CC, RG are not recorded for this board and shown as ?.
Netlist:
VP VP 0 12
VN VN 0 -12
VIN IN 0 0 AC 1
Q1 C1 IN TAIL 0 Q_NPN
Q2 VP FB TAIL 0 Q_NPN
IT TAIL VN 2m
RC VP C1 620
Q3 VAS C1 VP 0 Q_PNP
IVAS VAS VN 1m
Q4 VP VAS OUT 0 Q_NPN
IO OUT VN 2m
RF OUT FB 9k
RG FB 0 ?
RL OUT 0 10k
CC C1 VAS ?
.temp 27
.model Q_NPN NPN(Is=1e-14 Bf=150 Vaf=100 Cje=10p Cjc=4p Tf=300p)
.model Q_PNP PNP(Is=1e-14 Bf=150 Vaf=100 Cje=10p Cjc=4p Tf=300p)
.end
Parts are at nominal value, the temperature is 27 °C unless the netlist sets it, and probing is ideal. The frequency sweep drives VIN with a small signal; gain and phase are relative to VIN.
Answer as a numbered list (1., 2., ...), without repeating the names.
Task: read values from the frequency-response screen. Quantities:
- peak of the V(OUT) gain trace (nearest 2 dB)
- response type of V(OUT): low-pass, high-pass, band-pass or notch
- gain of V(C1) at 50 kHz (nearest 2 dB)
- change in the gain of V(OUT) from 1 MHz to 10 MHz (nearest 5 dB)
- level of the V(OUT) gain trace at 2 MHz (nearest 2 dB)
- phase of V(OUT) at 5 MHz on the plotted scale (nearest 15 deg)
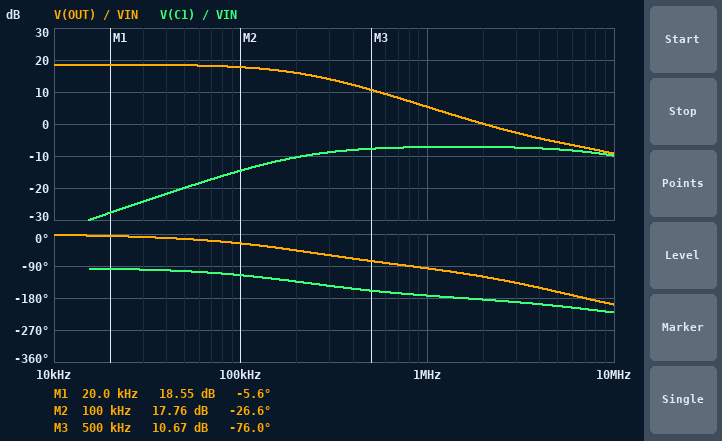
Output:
1. 18 dB
2. low-pass
3. -20 dB
4. -15 dB
5. 0 dB
6. -165 deg
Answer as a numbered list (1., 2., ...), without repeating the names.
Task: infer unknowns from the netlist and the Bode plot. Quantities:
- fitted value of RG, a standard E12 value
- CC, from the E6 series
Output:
1. 1.2 kΩ
2. 1.5 nF
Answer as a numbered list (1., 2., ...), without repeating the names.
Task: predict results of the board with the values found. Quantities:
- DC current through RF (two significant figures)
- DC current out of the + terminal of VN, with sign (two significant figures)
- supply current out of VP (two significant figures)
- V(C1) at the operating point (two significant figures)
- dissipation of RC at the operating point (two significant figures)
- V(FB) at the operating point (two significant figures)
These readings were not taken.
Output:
1. 2.6 µA
2. -5.0 mA
3. 5.0 mA
4. 11 V
5. 690 µW
6. -3.5 mV
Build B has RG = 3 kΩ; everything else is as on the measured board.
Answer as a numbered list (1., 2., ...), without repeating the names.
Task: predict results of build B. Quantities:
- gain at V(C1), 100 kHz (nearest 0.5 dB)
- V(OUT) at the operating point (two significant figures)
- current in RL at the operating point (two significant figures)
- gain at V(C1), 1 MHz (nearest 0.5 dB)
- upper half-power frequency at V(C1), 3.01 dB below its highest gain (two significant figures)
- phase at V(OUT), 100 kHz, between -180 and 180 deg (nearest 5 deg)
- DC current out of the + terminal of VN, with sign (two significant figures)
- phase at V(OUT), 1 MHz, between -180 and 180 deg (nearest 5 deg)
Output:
1. -20.5 dB
2. 36 mV
3. 3.6 µA
4. -8.0 dB
5. 5.6 MHz
6. -15 deg
7. -5.0 mA
8. -90 deg
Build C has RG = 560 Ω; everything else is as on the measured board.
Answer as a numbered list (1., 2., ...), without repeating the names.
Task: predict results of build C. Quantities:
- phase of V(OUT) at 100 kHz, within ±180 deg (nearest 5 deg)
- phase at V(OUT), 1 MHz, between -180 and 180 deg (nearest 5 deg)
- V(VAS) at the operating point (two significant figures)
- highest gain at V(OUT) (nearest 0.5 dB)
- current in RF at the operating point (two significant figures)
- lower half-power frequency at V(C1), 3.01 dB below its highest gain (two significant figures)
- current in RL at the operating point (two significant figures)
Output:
1. -45 deg
2. -100 deg
3. 660 mV
4. 24.5 dB
5. 780 nA
6. 110 kHz
7. 1.1 µA
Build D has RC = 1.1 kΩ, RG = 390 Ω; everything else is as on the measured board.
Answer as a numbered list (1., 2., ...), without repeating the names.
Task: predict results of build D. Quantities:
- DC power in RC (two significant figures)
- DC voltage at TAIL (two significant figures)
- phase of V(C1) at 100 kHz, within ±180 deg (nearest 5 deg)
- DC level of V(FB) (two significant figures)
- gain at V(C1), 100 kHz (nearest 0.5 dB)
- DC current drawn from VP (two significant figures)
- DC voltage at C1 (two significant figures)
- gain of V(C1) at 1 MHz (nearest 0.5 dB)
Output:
1. 390 µW
2. -640 mV
3. -145 deg
4. 22 mV
5. -9.5 dB
6. 5.1 mA
7. 11 V
8. -8.0 dB
